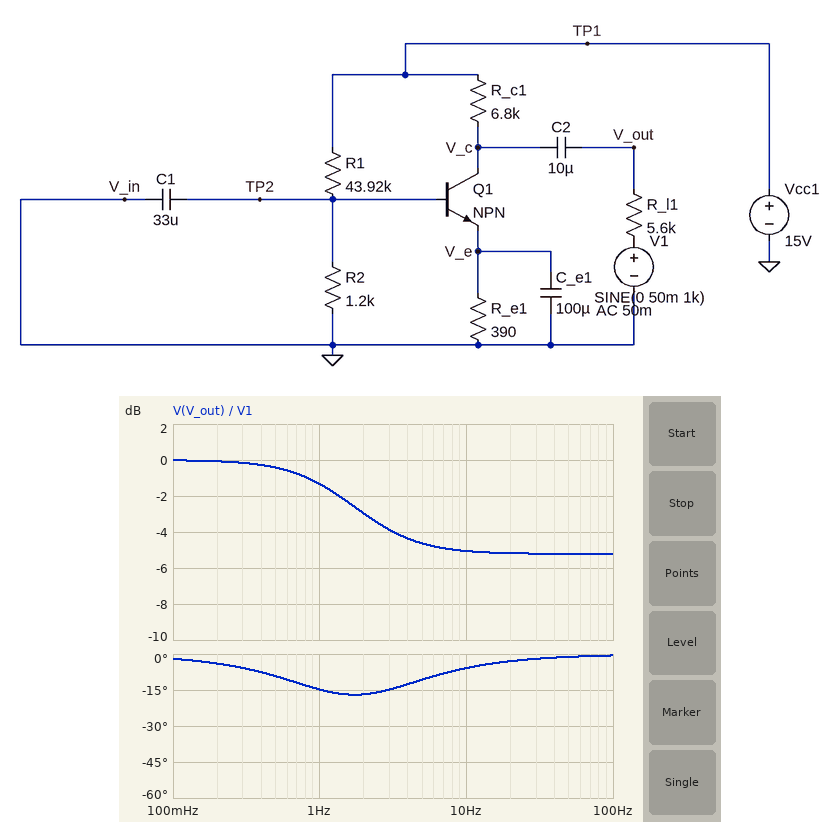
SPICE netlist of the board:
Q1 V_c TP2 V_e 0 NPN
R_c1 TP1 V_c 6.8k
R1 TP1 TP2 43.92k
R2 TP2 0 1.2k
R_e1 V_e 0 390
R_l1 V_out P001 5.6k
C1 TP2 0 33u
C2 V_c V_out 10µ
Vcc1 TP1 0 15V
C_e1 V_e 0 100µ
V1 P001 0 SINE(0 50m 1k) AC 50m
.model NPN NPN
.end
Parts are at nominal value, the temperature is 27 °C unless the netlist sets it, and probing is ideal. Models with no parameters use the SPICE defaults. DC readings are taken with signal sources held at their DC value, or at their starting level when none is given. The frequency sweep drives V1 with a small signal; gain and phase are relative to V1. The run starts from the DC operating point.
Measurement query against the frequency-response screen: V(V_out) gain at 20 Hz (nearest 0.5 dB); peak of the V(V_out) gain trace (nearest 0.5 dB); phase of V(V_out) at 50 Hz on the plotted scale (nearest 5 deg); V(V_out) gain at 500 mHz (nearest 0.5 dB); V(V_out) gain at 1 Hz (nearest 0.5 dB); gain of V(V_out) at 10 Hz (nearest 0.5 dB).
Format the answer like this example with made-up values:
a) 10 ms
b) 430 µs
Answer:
a) -5.0 dB
b) 0 dB
c) 0 deg
d) -0.5 dB
e) -1.5 dB
f) -5.0 dB
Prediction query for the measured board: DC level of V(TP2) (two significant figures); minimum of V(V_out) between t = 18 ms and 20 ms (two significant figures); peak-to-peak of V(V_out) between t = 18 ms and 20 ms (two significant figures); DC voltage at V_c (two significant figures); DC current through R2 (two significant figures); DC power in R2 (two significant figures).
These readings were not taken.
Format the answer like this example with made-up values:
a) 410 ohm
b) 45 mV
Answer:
a) 400 mV
b) -27 mV
c) 55 mV
d) 15 V
e) 330 µA
f) 130 µW
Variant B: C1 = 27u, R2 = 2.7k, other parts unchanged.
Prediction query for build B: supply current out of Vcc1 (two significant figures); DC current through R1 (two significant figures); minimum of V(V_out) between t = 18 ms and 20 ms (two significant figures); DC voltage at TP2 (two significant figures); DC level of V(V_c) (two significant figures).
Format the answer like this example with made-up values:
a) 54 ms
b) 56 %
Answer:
a) 620 µA
b) 320 µA
c) -27 mV
d) 860 mV
e) 13 V
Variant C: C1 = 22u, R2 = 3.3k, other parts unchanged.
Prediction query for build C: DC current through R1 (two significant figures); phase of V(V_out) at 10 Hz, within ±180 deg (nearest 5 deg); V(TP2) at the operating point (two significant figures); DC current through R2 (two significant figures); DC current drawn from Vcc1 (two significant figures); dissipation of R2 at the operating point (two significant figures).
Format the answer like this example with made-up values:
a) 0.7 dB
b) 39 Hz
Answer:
a) 320 µA
b) -5 deg
c) 1.0 V
d) 310 µA
e) 990 µA
f) 320 µW
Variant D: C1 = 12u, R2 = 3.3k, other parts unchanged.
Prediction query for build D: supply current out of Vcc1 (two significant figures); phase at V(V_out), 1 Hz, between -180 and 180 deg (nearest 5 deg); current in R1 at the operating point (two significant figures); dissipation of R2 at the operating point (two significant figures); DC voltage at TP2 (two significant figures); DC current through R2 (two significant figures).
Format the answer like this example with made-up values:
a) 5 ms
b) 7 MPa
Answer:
a) 990 µA
b) -15 deg
c) 320 µA
d) 320 µW
e) 1.0 V
f) 310 µA
